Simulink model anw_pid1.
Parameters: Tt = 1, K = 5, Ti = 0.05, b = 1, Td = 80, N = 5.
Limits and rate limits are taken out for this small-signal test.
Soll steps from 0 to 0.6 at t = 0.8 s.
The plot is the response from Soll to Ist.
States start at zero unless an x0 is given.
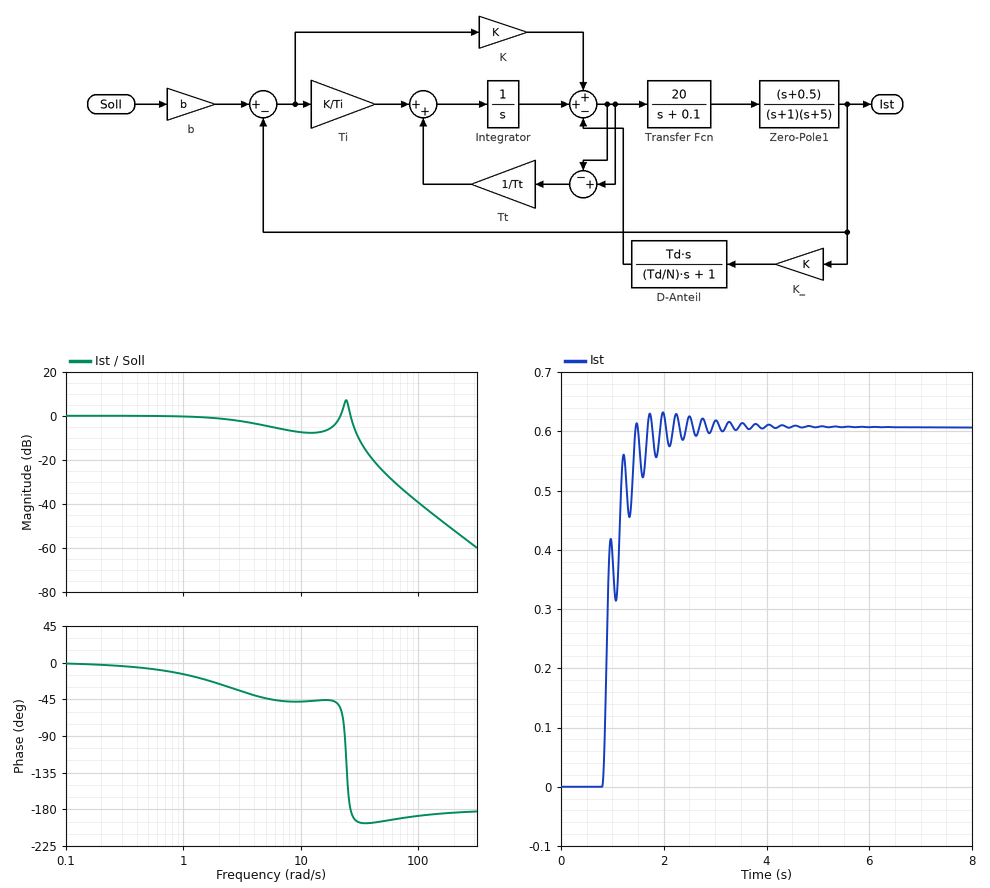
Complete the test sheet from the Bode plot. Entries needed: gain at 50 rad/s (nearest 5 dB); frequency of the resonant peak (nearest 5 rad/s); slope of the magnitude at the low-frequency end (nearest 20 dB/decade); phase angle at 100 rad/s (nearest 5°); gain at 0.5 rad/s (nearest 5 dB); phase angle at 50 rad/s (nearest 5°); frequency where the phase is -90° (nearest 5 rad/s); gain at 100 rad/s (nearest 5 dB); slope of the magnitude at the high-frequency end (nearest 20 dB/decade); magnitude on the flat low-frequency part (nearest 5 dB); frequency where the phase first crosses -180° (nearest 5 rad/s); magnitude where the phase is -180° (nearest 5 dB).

-25 dB
25 rad/s
0 dB/decade
-190°
0 dB
-195°
25 rad/s
-40 dB
-40 dB/decade
0 dB
25 rad/s
0 dB
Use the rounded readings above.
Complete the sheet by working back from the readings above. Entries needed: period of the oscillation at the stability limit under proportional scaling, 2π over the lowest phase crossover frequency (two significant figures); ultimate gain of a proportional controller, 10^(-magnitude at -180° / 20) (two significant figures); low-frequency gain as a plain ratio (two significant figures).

0.25 s
1.0
1.0
